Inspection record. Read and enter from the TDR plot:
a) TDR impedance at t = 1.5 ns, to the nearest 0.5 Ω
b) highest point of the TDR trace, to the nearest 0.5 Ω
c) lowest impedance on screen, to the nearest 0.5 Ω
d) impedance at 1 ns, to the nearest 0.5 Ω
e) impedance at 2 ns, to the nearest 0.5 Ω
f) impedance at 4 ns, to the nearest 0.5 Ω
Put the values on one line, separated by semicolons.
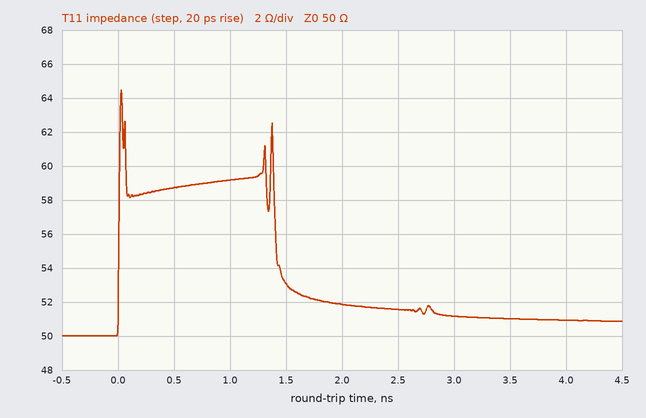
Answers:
53.0 Ω; 64.5 Ω; 50.0 Ω; 59.0 Ω; 52.0 Ω; 51.0 Ω
